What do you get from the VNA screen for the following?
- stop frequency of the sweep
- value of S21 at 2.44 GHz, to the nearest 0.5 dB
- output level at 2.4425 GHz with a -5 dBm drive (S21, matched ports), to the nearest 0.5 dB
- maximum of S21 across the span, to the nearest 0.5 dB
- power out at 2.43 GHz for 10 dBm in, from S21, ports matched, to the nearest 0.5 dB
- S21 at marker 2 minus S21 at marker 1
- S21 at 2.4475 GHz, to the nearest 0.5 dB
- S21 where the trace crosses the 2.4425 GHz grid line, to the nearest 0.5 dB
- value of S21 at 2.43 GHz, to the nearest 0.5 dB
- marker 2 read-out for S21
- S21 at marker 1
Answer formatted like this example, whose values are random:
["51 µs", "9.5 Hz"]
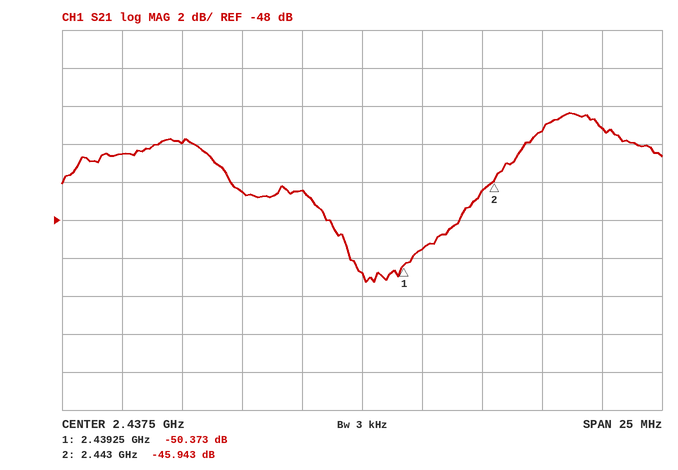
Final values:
["2.45 GHz", "-49.5 dB", "-51.5 dBm", "-42.5 dB", "-34.0 dBm", "4.430 dB", "-43.0 dB", "-46.5 dB", "-44.0 dB", "-45.943 dB", "-50.373 dB"]
